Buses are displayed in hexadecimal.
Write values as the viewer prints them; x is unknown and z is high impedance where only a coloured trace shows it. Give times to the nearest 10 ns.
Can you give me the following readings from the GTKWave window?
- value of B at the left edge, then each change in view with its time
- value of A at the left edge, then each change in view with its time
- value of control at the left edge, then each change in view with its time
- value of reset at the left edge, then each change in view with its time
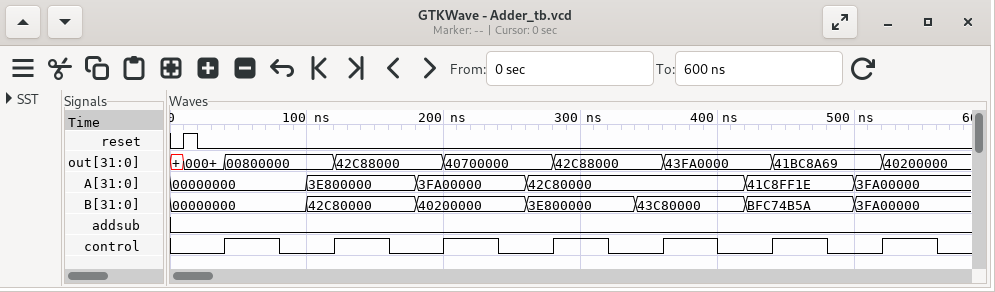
00000000, 42C80000 at 100 ns, 40200000 at 180 ns, 3E800000 at 260 ns, 43C80000 at 340 ns, BFC74B5A at 420 ns, 3FA00000 at 500 ns
00000000, 3E800000 at 100 ns, 3FA00000 at 180 ns, 42C80000 at 260 ns, 41C8FF1E at 420 ns, 3FA00000 at 500 ns
0, 1 at 40 ns, 0 at 80 ns, 1 at 120 ns, 0 at 160 ns, 1 at 200 ns, 0 at 240 ns, 1 at 280 ns, 0 at 320 ns, 1 at 360 ns, 0 at 400 ns, 1 at 440 ns, 0 at 480 ns, 1 at 520 ns, 0 at 560 ns
0, 1 at 10 ns, 0 at 20 ns
